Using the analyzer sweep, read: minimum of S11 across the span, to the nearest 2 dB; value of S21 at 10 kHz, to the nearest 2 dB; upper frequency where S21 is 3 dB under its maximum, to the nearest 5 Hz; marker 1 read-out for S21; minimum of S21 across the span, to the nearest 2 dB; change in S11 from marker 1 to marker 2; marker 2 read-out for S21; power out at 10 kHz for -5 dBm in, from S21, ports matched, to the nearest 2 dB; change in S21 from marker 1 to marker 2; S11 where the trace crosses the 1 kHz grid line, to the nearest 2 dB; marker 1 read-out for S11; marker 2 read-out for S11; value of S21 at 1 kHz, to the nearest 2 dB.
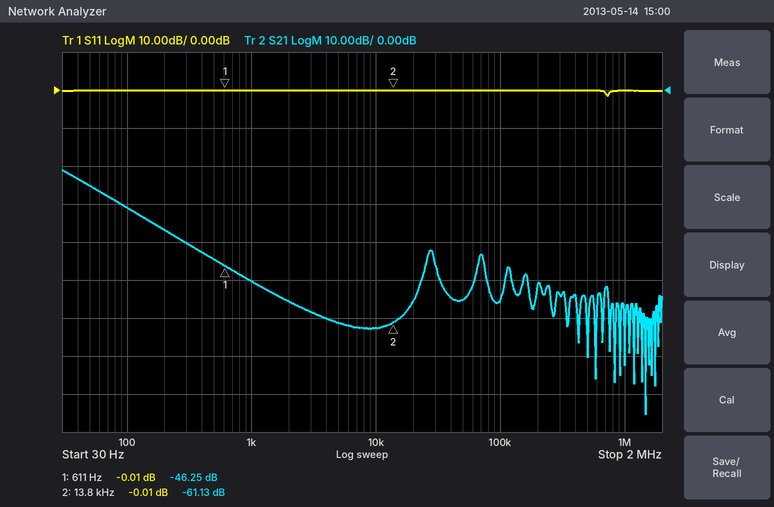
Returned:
-2 dB
-62 dB
45 Hz
-46.25 dB
-86 dB
0.00 dB
-61.13 dB
-68 dBm
-14.88 dB
0 dB
-0.01 dB
-0.01 dB
-50 dB
